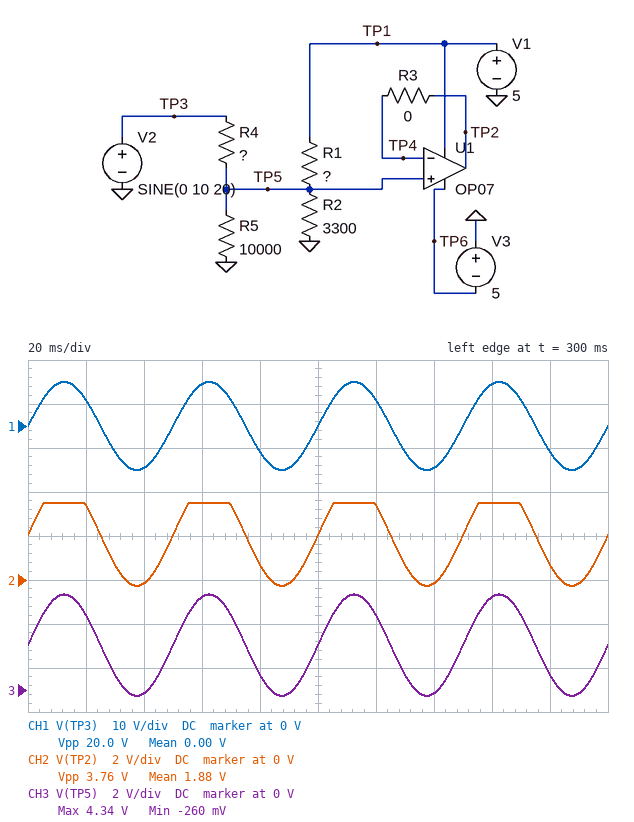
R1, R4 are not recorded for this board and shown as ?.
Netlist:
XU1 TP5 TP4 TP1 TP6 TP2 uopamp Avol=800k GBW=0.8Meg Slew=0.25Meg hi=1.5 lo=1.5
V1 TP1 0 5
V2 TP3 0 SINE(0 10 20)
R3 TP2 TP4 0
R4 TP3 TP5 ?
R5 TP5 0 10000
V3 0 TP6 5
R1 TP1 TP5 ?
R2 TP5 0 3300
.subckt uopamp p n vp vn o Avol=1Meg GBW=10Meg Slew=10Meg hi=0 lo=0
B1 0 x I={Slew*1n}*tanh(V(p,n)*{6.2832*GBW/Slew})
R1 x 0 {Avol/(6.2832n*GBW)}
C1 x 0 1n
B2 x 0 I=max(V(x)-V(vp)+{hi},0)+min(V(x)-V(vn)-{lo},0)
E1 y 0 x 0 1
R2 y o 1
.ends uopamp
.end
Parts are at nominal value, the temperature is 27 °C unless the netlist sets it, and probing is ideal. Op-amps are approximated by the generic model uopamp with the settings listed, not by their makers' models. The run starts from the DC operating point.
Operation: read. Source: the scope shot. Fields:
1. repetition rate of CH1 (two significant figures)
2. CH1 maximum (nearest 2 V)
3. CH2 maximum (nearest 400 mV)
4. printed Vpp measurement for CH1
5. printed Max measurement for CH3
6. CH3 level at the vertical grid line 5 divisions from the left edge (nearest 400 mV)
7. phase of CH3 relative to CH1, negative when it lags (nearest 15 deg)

20 Hz
10 V
3.6 V
20.0 V
4.34 V
2.0 V
0 deg
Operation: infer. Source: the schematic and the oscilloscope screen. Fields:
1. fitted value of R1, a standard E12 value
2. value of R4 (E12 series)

2.2 kΩ
3.9 kΩ
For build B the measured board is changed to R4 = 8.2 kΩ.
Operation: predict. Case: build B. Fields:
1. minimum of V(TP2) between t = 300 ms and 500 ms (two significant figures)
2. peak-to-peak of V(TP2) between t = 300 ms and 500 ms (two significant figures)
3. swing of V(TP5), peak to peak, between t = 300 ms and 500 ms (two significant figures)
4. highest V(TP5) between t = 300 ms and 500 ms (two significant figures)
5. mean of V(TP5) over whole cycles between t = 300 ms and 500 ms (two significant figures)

1.1 V
2.4 V
2.5 V
3.6 V
2.3 V
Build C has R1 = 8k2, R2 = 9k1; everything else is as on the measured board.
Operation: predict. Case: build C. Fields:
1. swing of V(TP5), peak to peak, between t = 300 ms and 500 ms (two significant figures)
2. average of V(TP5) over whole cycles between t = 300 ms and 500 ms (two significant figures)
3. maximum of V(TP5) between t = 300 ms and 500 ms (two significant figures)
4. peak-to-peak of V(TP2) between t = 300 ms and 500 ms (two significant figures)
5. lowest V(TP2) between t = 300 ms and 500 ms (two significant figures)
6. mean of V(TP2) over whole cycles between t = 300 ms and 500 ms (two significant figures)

8.7 V
1.0 V
5.4 V
6.8 V
-3.3 V
650 mV
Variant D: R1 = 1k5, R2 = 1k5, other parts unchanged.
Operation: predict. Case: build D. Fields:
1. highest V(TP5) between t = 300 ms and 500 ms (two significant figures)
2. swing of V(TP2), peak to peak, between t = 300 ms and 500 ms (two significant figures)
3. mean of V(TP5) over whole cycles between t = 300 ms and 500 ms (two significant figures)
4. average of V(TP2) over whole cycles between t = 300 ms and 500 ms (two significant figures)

3.5 V
3.0 V
2.0 V
2.0 V
